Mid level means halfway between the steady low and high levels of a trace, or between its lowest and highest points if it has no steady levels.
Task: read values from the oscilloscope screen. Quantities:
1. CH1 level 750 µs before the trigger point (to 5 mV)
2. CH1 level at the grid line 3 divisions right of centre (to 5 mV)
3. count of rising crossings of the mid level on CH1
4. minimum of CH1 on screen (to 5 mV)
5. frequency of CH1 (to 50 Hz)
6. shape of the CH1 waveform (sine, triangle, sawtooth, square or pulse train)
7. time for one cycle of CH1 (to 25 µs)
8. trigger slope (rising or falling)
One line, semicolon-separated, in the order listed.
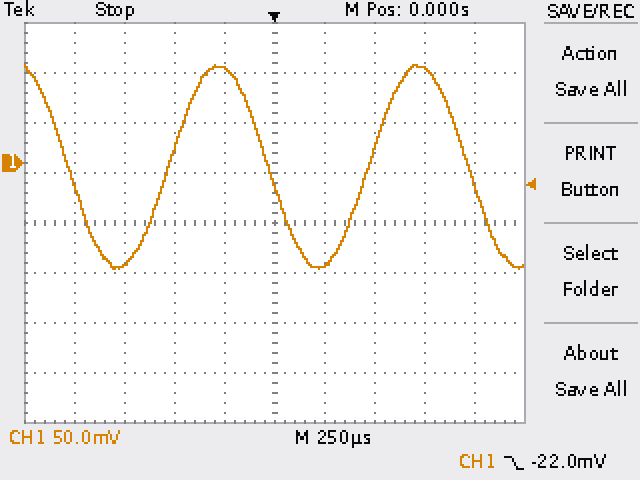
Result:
-100 mV; 95 mV; 2; -105 mV; 1.00 kHz; sine; 1.000 ms; falling
